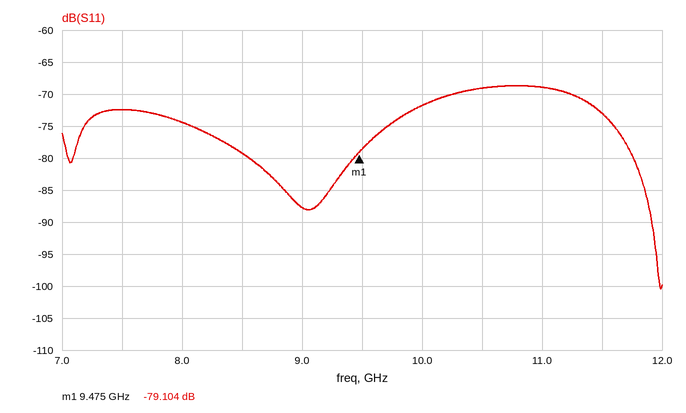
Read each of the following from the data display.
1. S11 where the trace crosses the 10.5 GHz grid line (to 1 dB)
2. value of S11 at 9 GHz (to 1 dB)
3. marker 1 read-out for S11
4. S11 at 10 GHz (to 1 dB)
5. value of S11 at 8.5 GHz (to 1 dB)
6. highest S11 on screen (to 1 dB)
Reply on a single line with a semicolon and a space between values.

-69 dB; -88 dB; -79.104 dB; -72 dB; -79 dB; -69 dB
